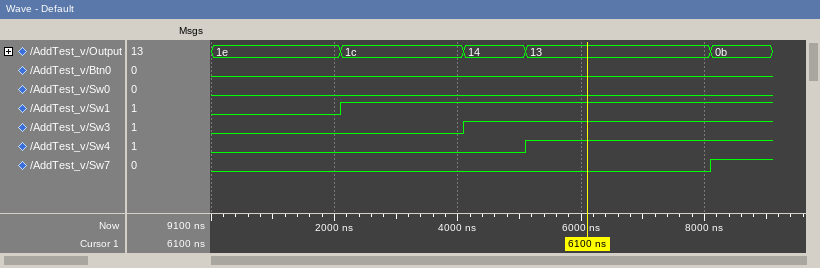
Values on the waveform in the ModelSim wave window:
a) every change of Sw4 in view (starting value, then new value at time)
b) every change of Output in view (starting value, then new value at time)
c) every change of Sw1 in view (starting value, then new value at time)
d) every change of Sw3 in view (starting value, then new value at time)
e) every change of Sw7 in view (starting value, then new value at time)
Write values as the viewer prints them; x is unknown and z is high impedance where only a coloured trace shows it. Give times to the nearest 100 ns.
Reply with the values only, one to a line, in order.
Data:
0, 1 at 5100 ns
1e, 1c at 2100 ns, 14 at 4100 ns, 13 at 5100 ns, 0b at 8100 ns
0, 1 at 2100 ns
0, 1 at 4100 ns
0, 1 at 8100 ns
